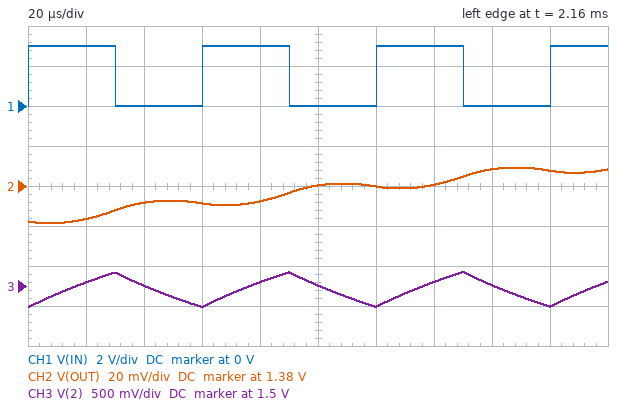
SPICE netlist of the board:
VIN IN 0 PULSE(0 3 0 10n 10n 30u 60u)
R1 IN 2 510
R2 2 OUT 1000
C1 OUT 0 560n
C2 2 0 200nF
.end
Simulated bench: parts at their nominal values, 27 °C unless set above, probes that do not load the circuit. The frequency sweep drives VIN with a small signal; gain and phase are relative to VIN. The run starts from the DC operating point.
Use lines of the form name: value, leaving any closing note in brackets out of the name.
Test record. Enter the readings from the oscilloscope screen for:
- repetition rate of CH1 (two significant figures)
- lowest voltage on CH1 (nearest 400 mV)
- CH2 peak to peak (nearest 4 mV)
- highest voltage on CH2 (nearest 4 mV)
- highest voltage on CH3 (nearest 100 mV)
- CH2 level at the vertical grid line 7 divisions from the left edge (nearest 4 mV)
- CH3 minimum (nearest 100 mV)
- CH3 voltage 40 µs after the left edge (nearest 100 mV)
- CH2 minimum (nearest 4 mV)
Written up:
repetition rate of CH1: 17 kHz
lowest voltage on CH1: 0 V
CH2 peak to peak: 28 mV
highest voltage on CH2: 1.388 V
highest voltage on CH3: 1.7 V
CH2 level at the vertical grid line 7 divisions from the left edge: 1.380 V
CH3 minimum: 1.2 V
CH3 voltage 40 µs after the left edge: 1.5 V
CH2 minimum: 1.360 V
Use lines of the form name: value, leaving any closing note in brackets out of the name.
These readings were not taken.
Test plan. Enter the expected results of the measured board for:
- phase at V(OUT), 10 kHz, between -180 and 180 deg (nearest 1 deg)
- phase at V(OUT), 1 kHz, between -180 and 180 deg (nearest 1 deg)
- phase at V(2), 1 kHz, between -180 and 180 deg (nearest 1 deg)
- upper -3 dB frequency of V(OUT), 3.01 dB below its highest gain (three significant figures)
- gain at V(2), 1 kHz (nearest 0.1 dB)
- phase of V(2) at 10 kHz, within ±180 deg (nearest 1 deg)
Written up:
phase at V(OUT), 10 kHz, between -180 and 180 deg: -165 deg
phase at V(OUT), 1 kHz, between -180 and 180 deg: -102 deg
phase at V(2), 1 kHz, between -180 and 180 deg: -28 deg
upper -3 dB frequency of V(OUT), 3.01 dB below its highest gain: 179 Hz
gain at V(2), 1 kHz: -4.4 dB
phase of V(2) at 10 kHz, within ±180 deg: -77 deg
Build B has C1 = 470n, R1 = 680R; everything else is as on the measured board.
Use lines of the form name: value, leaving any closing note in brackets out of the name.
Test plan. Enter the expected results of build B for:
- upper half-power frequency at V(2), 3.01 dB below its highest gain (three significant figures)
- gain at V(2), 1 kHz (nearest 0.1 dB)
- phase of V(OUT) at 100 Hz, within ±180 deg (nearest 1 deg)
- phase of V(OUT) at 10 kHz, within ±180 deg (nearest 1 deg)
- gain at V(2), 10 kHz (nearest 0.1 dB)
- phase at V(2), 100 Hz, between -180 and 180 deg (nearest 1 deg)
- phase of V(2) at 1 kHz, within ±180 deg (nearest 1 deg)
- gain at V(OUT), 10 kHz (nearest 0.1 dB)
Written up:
upper half-power frequency at V(2), 3.01 dB below its highest gain: 290 Hz
gain at V(2), 1 kHz: -5.7 dB
phase of V(OUT) at 100 Hz, within ±180 deg: -31 deg
phase of V(OUT) at 10 kHz, within ±180 deg: -167 deg
gain at V(2), 10 kHz: -18.8 dB
phase at V(2), 100 Hz, between -180 and 180 deg: -14 deg
phase of V(2) at 1 kHz, within ±180 deg: -33 deg
gain at V(OUT), 10 kHz: -48.2 dB
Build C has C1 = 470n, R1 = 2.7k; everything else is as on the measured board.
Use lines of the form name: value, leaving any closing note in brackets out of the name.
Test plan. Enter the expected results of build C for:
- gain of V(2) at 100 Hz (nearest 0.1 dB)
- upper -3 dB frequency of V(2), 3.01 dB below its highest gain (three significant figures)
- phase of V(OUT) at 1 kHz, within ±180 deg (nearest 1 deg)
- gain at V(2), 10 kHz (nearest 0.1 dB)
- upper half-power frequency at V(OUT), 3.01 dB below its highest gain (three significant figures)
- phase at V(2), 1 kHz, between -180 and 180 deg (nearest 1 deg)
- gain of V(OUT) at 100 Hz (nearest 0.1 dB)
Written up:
gain of V(2) at 100 Hz: -4.2 dB
upper -3 dB frequency of V(2), 3.01 dB below its highest gain: 77.1 Hz
phase of V(OUT) at 1 kHz, within ±180 deg: -122 deg
gain at V(2), 10 kHz: -30.7 dB
upper half-power frequency at V(OUT), 3.01 dB below its highest gain: 73.4 Hz
phase at V(2), 1 kHz, between -180 and 180 deg: -51 deg
gain of V(OUT) at 100 Hz: -4.6 dB
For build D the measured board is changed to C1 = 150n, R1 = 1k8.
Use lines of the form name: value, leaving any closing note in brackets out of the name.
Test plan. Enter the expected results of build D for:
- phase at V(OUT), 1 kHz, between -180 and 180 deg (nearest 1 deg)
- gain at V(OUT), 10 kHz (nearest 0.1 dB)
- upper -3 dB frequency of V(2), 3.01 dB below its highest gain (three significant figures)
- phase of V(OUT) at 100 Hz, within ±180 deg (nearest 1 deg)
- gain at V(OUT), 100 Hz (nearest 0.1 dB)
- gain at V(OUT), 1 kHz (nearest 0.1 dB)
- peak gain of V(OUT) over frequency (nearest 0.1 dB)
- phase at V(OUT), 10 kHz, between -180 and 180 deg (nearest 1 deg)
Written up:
phase at V(OUT), 1 kHz, between -180 and 180 deg: -103 deg
gain at V(OUT), 10 kHz: -46.8 dB
upper -3 dB frequency of V(2), 3.01 dB below its highest gain: 234 Hz
phase of V(OUT) at 100 Hz, within ±180 deg: -27 deg
gain at V(OUT), 100 Hz: -0.8 dB
gain at V(OUT), 1 kHz: -14.0 dB
peak gain of V(OUT) over frequency: 0 dB
phase at V(OUT), 10 kHz, between -180 and 180 deg: -167 deg
